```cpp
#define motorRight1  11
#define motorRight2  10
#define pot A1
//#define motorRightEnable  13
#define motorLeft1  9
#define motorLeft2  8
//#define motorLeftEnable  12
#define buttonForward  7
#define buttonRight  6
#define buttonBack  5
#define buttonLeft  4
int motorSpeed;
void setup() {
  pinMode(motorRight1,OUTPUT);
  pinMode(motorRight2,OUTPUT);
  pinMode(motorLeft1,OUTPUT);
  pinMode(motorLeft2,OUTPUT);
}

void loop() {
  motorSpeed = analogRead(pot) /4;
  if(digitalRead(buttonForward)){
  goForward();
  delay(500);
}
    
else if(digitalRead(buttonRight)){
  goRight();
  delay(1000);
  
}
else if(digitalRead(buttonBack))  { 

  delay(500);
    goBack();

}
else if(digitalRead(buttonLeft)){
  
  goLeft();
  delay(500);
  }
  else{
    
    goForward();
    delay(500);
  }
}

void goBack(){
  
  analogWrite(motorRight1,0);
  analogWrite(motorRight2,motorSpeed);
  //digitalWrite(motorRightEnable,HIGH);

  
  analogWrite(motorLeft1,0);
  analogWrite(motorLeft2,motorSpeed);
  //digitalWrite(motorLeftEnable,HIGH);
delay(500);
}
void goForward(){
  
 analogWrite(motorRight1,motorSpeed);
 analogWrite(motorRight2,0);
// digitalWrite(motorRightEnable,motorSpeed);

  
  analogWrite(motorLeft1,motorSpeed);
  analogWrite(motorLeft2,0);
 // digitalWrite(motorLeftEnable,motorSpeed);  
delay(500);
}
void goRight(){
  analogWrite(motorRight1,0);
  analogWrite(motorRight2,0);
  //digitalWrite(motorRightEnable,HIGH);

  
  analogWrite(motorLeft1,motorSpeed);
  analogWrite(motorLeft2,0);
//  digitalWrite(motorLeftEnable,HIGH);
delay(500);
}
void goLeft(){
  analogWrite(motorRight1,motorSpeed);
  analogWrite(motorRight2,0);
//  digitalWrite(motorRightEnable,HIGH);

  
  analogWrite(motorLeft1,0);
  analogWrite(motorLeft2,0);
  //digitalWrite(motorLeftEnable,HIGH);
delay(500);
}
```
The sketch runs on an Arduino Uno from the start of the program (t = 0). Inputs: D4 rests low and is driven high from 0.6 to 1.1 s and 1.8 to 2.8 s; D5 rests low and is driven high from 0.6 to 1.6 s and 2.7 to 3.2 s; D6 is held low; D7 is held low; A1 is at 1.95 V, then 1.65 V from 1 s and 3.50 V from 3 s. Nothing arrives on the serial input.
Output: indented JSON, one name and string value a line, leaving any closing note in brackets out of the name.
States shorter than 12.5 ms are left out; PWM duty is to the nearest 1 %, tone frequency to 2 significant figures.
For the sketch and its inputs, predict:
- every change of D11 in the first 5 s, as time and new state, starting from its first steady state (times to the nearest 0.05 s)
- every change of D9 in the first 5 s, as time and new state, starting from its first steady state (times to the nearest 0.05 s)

{
  "every change of D11 in the first 5 s, as time and new state, starting from its first steady state": "0 s PWM 39 %; 1.5 s low; 2 s PWM 33 %; 3.5 s low; 4 s PWM 70 %",
  "every change of D9 in the first 5 s, as time and new state, starting from its first steady state": "0 s PWM 39 %; 1.5 s low; 4 s PWM 70 %"
}
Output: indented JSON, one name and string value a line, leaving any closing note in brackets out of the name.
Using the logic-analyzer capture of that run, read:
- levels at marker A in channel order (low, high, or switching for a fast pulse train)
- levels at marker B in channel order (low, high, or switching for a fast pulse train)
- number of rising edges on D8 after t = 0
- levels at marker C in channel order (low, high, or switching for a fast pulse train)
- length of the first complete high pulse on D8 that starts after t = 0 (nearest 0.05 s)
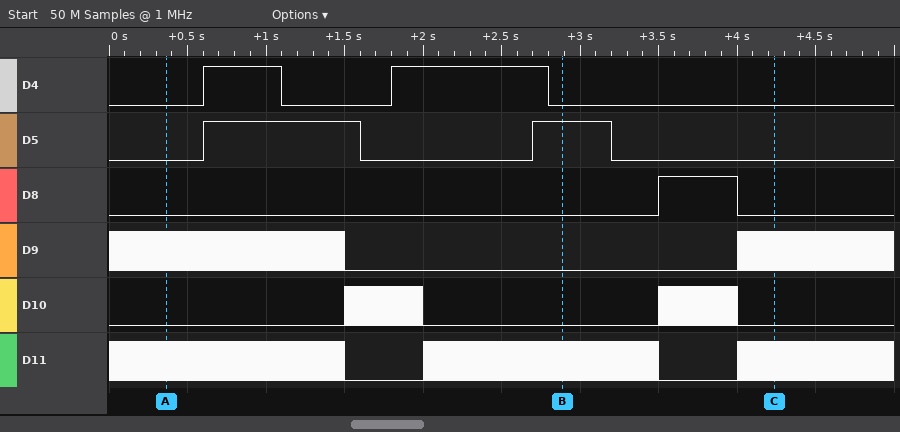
{
  "levels at marker A in channel order": "D4 low, D5 low, D8 low, D9 switching, D10 low, D11 switching",
  "levels at marker B in channel order": "D4 low, D5 high, D8 low, D9 low, D10 low, D11 switching",
  "number of rising edges on D8 after t = 0": "1",
  "levels at marker C in channel order": "D4 low, D5 low, D8 low, D9 switching, D10 low, D11 switching",
  "length of the first complete high pulse on D8 that starts after t = 0": "0.50 s"
}
